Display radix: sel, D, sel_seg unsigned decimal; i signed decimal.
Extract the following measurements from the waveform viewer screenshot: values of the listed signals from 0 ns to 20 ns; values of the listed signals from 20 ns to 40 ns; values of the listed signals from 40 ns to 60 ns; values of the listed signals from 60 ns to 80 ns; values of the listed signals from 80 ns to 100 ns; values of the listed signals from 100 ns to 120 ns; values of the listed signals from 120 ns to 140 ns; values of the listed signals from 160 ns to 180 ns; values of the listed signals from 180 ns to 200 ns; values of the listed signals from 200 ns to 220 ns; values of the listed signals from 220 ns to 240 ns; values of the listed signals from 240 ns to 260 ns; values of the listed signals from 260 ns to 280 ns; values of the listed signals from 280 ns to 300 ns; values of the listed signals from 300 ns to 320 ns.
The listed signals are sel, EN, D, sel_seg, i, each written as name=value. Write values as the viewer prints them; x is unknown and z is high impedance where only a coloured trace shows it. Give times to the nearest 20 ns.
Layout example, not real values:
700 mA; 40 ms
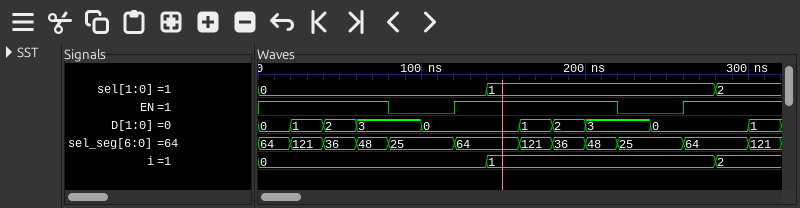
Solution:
sel=0, EN=1, D=0, sel_seg=64, i=0; sel=0, EN=1, D=1, sel_seg=121, i=0; sel=0, EN=1, D=2, sel_seg=36, i=0; sel=0, EN=1, D=3, sel_seg=48, i=0; sel=0, EN=0, D=3, sel_seg=25, i=0; sel=0, EN=0, D=0, sel_seg=25, i=0; sel=0, EN=1, D=0, sel_seg=64, i=0; sel=1, EN=1, D=1, sel_seg=121, i=1; sel=1, EN=1, D=2, sel_seg=36, i=1; sel=1, EN=1, D=3, sel_seg=48, i=1; sel=1, EN=0, D=3, sel_seg=25, i=1; sel=1, EN=0, D=0, sel_seg=25, i=1; sel=1, EN=1, D=0, sel_seg=64, i=1; sel=2, EN=1, D=0, sel_seg=64, i=2; sel=2, EN=1, D=1, sel_seg=121, i=2
